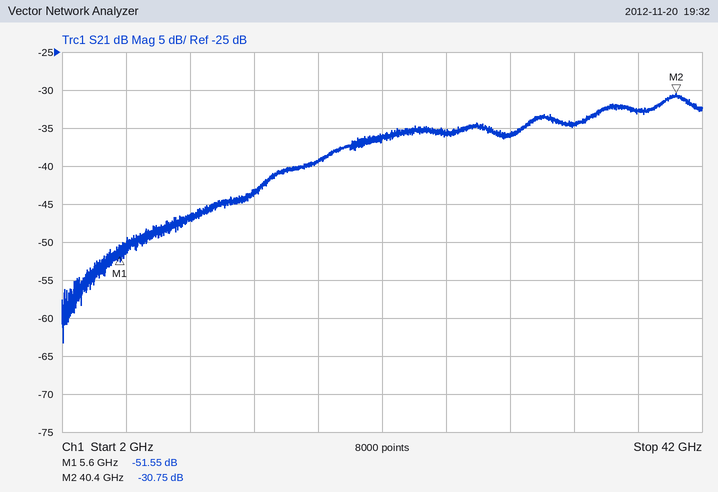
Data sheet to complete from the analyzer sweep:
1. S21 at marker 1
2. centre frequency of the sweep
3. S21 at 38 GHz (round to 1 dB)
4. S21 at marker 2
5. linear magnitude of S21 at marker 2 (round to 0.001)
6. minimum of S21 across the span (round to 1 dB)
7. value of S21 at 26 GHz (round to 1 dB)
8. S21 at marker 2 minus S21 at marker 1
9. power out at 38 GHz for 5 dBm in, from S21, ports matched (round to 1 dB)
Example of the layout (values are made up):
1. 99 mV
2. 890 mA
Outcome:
1. -51.55 dB
2. 22 GHz
3. -33 dB
4. -30.75 dB
5. 0.029
6. -63 dB
7. -36 dB
8. 20.80 dB
9. -28 dBm
